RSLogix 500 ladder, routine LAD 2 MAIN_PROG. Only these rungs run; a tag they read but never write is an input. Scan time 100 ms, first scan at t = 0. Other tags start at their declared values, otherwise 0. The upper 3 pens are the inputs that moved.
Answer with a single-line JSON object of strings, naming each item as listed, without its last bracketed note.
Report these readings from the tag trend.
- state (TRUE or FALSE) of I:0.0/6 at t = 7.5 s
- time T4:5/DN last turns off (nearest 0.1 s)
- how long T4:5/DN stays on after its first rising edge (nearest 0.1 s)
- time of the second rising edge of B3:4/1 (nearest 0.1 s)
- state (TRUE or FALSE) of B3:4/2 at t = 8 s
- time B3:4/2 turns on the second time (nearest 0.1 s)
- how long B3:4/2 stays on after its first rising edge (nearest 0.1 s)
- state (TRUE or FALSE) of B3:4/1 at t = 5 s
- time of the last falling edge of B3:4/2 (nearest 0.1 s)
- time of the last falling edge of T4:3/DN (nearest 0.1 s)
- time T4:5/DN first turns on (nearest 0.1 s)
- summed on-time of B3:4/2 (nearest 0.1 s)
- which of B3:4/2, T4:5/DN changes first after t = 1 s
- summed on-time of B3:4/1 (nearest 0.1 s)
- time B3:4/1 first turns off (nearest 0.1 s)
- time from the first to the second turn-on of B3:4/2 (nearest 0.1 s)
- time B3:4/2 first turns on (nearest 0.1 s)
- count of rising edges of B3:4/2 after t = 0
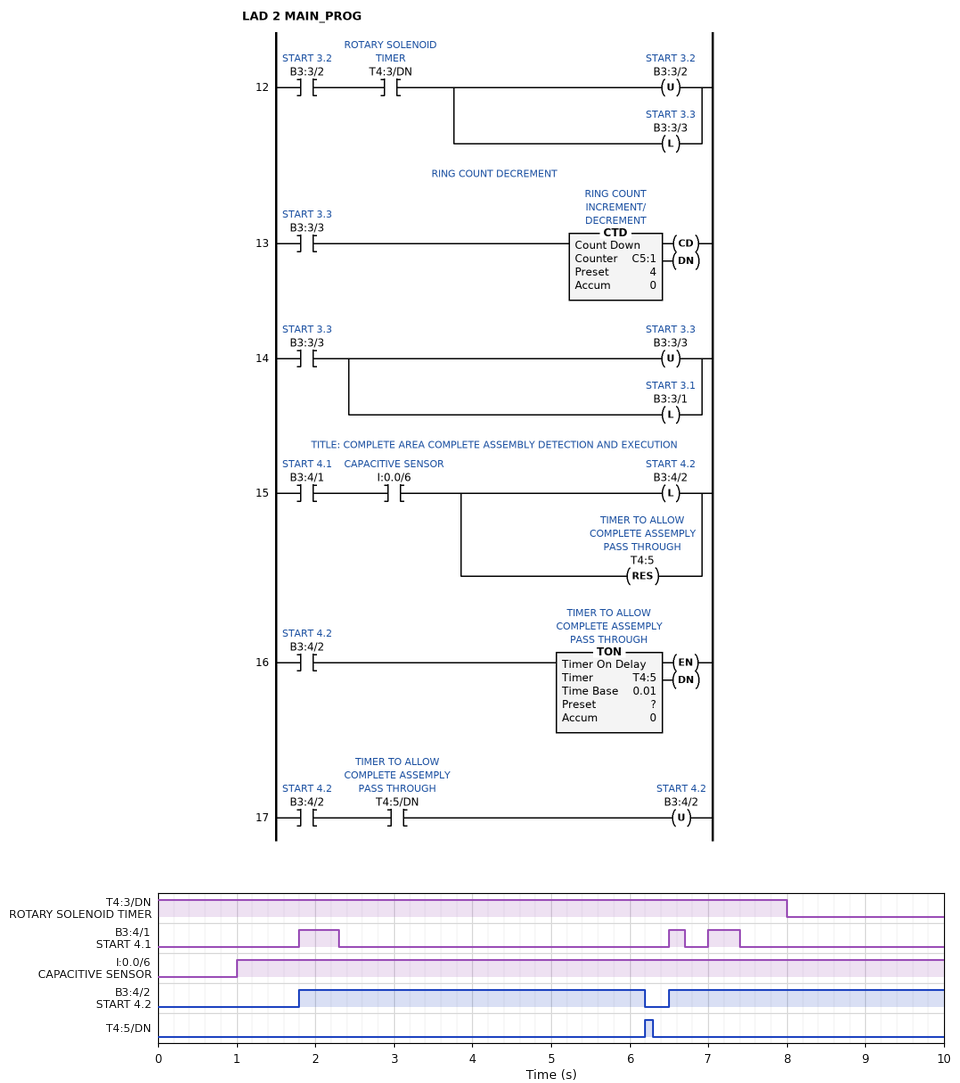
{"state (TRUE or FALSE) of I:0.0/6 at t = 7.5 s": "TRUE", "time T4:5/DN last turns off": "6.3 s", "how long T4:5/DN stays on after its first rising edge": "0.1 s", "time of the second rising edge of B3:4/1": "6.5 s", "state (TRUE or FALSE) of B3:4/2 at t = 8 s": "TRUE", "time B3:4/2 turns on the second time": "6.5 s", "how long B3:4/2 stays on after its first rising edge": "4.4 s", "state (TRUE or FALSE) of B3:4/1 at t = 5 s": "FALSE", "time of the last falling edge of B3:4/2": "6.2 s", "time of the last falling edge of T4:3/DN": "8.0 s", "time T4:5/DN first turns on": "6.2 s", "summed on-time of B3:4/2": "7.9 s", "which of B3:4/2, T4:5/DN changes first after t = 1 s": "B3:4/2", "summed on-time of B3:4/1": "1.1 s", "time B3:4/1 first turns off": "2.3 s", "time from the first to the second turn-on of B3:4/2": "4.7 s", "time B3:4/2 first turns on": "1.8 s", "count of rising edges of B3:4/2 after t = 0": "2"}
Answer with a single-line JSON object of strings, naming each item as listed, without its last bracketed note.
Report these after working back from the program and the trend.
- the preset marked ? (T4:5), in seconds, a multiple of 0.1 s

{"the preset marked ? (T4:5), in seconds, a multiple of 0.1 s": "4.0 s"}
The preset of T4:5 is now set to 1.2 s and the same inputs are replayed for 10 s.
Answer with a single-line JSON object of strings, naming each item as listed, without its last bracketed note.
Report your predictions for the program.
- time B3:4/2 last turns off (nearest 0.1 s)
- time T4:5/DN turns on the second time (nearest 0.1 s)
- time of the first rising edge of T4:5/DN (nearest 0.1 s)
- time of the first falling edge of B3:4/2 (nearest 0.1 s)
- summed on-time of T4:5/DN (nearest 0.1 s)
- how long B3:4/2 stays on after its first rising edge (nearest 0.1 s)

{"time B3:4/2 last turns off": "8.5 s", "time T4:5/DN turns on the second time": "8.5 s", "time of the first rising edge of T4:5/DN": "3.4 s", "time of the first falling edge of B3:4/2": "3.4 s", "summed on-time of T4:5/DN": "0.2 s", "how long B3:4/2 stays on after its first rising edge": "1.6 s"}
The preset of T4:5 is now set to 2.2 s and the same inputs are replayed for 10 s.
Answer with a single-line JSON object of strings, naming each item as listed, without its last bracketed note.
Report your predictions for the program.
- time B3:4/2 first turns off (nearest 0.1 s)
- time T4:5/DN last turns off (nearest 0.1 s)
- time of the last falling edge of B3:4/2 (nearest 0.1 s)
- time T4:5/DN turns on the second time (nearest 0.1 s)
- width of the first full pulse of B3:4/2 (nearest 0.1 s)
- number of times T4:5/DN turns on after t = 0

{"time B3:4/2 first turns off": "4.4 s", "time T4:5/DN last turns off": "9.6 s", "time of the last falling edge of B3:4/2": "9.5 s", "time T4:5/DN turns on the second time": "9.5 s", "width of the first full pulse of B3:4/2": "2.6 s", "number of times T4:5/DN turns on after t = 0": "2"}
